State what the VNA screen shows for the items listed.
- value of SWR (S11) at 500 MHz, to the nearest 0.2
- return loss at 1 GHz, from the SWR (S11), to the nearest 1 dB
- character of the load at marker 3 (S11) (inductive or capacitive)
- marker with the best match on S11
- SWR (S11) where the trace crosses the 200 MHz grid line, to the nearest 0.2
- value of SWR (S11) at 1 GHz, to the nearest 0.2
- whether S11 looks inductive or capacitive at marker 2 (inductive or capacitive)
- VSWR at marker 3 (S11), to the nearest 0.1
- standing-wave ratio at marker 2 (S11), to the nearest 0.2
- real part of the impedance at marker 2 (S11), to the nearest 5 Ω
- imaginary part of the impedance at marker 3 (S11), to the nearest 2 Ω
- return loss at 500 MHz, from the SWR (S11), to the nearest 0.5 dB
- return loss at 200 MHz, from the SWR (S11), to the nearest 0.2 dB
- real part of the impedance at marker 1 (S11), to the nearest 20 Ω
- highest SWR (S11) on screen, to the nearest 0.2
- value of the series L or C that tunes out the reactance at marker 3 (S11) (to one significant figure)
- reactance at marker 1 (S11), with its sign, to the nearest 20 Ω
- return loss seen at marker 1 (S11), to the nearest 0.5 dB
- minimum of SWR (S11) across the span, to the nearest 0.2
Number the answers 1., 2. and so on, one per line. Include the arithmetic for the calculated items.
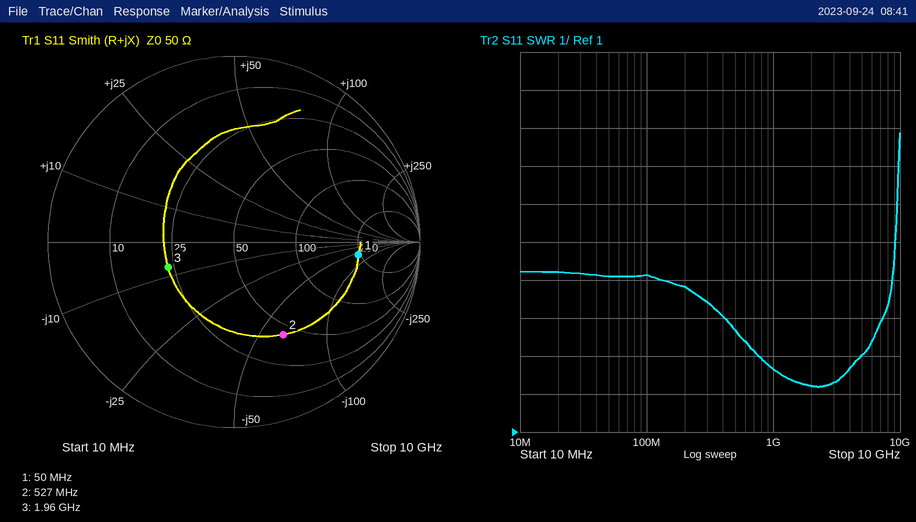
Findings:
1. 3.6
2. −20 log10((2.6 − 1)/(2.6 + 1)) ≈ 7 dB
3. capacitive
4. marker 3
5. 4.8
6. 2.6
7. capacitive
8. 2.2
9. 3.6
10. 45 Ω
11. -8 Ω
12. −20 log10((3.6 − 1)/(3.6 + 1)) ≈ 5.0 dB
13. −20 log10((4.8 − 1)/(4.8 + 1)) ≈ 3.67 dB, so 3.6 dB to the nearest 0.2 dB
14. 240 Ω
15. 8.8
16. L = 8 Ω/(2π × 1.96 GHz) ≈ 650 pH, so 600 pH to one significant figure
17. -60 Ω
18. 3.5 dB
19. 2.2
